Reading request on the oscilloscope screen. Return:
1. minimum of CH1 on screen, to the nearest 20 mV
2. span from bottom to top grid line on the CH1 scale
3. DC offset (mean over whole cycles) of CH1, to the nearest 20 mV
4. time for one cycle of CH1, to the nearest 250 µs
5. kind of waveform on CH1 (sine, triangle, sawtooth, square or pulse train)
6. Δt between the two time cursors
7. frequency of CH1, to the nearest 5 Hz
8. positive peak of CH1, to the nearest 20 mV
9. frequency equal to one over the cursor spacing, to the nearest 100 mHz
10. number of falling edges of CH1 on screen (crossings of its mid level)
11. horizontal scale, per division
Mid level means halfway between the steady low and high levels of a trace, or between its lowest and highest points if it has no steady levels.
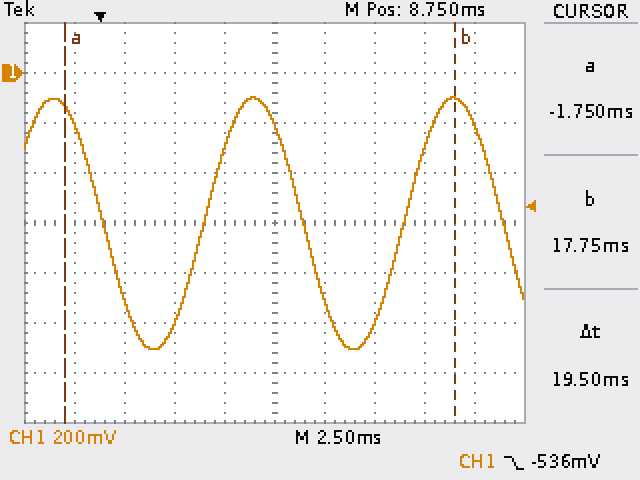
-1.10 V
1.6 V
-600 mV
10.00 ms
sine
19.5 ms
100 Hz
-100 mV
51.3 Hz
3
2.5 ms
